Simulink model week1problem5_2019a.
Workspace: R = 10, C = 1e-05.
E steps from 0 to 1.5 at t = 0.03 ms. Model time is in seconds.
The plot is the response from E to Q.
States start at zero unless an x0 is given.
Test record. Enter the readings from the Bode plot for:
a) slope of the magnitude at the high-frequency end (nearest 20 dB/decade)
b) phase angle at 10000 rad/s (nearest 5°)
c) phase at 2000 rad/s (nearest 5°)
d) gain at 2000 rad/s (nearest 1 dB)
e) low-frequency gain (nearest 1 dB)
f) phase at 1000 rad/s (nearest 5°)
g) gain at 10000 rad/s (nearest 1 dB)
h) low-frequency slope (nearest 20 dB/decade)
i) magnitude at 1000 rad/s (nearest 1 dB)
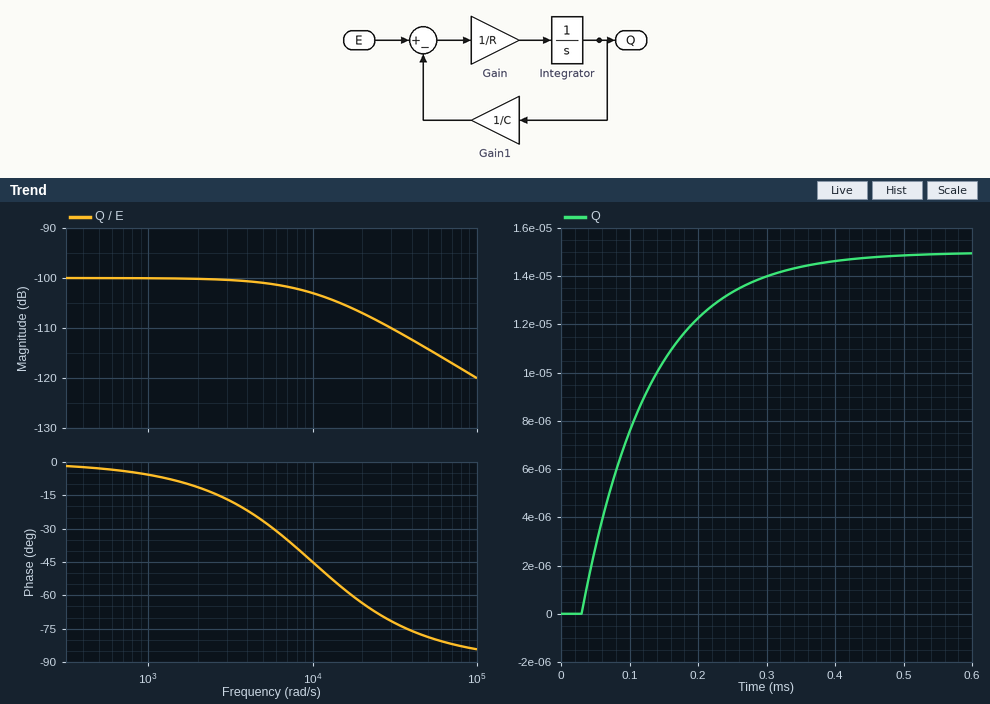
-20 dB/decade
-45°
-10°
-100 dB
-100 dB
-5°
-103 dB
0 dB/decade
-100 dB
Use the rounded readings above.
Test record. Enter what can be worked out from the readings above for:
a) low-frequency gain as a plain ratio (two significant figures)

0.000010
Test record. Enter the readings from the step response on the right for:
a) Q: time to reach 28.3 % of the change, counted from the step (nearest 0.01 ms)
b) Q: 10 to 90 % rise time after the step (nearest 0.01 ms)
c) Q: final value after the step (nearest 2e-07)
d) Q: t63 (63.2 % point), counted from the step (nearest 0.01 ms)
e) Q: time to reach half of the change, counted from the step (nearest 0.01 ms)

0.03 ms
0.22 ms
0.0000150
0.10 ms
0.07 ms
